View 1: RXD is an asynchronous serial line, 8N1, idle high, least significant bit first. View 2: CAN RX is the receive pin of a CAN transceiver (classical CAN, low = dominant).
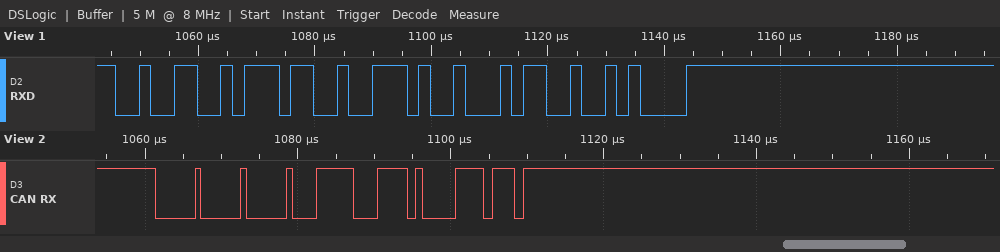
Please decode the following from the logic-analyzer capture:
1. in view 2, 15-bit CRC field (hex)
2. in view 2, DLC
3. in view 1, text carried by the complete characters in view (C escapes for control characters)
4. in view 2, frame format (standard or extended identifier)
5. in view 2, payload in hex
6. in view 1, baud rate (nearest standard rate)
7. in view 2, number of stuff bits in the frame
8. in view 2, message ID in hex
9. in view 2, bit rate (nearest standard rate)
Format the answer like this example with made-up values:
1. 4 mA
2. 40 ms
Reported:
1. 0x687B
2. 1
3. "27.4\n"
4. standard
5. F3
6. 500000 baud
7. 4
8. 0x000
9. 1000 kbit/s
